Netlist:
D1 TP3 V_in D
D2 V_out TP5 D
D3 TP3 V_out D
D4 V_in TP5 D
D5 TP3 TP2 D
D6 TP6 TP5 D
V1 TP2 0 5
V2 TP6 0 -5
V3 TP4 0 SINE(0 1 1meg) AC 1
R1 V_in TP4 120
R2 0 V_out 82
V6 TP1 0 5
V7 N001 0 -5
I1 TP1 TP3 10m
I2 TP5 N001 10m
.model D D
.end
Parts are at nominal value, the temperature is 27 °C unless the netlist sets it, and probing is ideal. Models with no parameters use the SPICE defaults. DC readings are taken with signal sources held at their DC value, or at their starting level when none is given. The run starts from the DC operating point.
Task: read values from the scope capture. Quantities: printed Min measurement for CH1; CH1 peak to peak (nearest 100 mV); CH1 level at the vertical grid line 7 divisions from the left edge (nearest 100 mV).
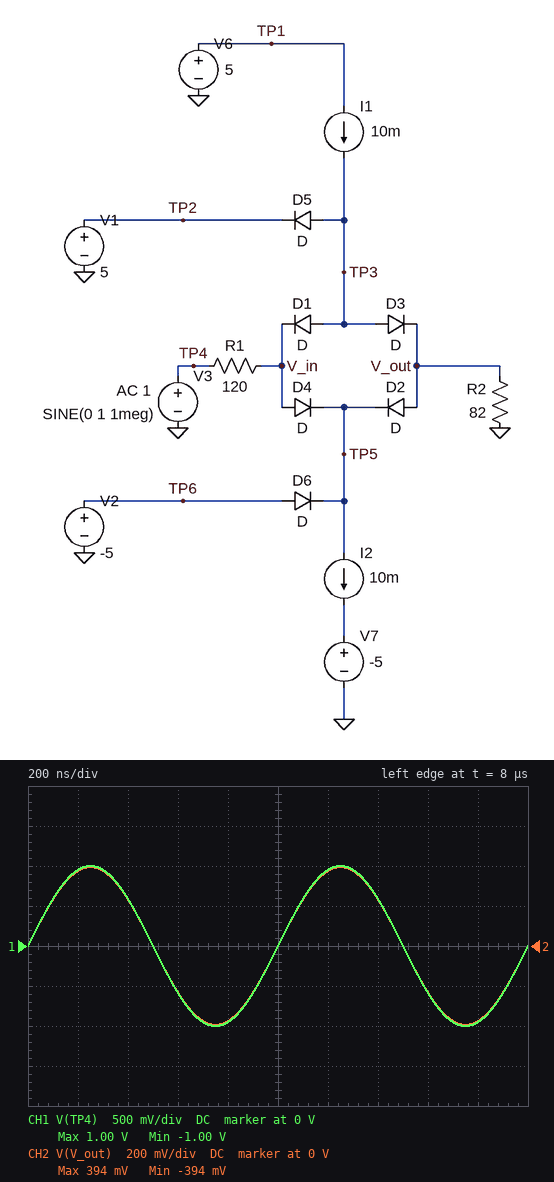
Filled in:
-1.00 V
2.0 V
600 mV
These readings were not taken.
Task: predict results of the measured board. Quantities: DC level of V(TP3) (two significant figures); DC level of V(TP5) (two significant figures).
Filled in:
700 mV
-700 mV
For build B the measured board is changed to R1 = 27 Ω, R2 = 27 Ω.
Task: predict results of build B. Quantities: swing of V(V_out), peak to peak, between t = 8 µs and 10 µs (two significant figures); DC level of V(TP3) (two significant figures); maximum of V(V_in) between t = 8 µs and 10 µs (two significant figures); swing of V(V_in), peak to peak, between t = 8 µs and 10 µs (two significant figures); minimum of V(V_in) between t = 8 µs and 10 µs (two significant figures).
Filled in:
540 mV
700 mV
730 mV
1.5 V
-730 mV
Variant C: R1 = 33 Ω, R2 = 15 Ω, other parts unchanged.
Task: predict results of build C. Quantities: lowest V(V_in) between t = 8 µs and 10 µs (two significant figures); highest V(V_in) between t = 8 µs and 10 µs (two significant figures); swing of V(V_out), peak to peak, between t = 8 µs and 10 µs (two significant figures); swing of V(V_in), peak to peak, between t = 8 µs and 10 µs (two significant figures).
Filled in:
-670 mV
670 mV
300 mV
1.3 V
